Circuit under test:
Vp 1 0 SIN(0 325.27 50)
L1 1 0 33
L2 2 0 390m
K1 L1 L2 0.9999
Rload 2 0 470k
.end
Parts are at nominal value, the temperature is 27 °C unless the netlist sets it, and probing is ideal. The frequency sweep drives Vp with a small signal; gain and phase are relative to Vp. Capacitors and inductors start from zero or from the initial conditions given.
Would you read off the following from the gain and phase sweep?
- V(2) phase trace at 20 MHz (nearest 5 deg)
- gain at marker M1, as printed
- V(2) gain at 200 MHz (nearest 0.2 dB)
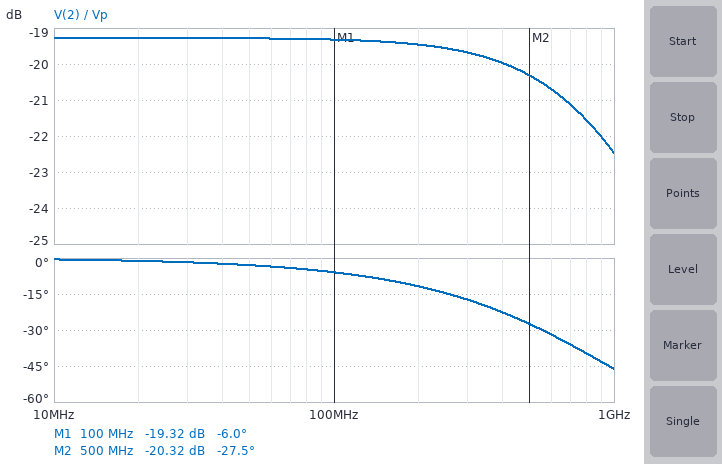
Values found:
0 deg
-19.32 dB
-19.4 dB
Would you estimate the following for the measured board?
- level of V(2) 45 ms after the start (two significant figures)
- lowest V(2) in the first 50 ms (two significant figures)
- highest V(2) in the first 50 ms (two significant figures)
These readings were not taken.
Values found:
35 V
-35 V
35 V
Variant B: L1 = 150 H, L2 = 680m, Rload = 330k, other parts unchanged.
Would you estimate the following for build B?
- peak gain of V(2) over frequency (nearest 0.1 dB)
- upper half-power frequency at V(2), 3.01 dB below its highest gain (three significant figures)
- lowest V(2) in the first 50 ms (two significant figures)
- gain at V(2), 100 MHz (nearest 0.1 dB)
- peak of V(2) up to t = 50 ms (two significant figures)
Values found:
-23.4 dB
386 MHz
-22 V
-23.7 dB
22 V
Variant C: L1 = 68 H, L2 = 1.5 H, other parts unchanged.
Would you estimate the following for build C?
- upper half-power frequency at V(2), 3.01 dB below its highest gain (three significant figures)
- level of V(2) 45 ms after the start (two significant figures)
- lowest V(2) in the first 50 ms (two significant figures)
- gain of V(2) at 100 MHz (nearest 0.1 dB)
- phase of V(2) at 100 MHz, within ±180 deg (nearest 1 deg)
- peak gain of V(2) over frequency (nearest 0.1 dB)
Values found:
249 MHz
48 V
-48 V
-17.2 dB
-22 deg
-16.6 dB
